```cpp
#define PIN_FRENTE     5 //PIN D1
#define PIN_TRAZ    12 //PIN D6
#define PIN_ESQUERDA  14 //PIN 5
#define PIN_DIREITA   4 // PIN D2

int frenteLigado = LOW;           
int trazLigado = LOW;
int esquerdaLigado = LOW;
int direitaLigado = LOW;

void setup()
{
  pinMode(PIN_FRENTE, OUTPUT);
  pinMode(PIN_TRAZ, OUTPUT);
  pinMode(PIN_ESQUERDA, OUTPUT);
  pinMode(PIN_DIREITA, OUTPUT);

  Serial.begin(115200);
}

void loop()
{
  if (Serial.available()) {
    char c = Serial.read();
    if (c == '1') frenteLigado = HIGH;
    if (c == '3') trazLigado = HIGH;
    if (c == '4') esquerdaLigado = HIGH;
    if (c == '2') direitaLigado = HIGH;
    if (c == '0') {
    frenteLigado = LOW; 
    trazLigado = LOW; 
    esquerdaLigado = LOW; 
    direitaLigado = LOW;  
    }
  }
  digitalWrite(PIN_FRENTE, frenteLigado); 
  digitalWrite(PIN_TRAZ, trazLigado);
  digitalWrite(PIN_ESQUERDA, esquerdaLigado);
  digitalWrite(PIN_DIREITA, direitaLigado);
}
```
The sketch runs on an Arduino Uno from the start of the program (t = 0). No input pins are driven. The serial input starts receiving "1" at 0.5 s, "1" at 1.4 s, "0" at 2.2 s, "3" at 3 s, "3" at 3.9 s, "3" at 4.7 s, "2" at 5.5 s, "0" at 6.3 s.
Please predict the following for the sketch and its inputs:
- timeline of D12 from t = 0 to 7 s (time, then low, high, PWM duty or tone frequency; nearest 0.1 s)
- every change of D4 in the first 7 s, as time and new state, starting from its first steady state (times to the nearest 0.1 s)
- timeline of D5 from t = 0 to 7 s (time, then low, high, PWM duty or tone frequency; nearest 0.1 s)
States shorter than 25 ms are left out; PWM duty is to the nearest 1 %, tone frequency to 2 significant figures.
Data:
0 s low; 3 s high; 6.3 s low
0 s low; 5.5 s high; 6.3 s low
0 s low; 0.5 s high; 2.2 s low
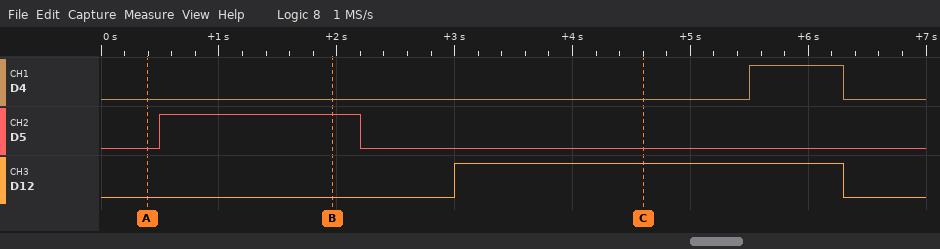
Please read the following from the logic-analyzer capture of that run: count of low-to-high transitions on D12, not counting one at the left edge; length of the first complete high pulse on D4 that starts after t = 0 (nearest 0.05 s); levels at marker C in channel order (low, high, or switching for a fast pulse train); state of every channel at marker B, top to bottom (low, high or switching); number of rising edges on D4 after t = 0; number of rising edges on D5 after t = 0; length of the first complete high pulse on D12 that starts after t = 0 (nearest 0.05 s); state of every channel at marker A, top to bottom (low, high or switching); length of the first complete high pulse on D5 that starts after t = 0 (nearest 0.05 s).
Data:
1
0.80 s
D4 low, D5 low, D12 high
D4 low, D5 high, D12 low
1
1
3.30 s
D4 low, D5 low, D12 low
1.70 s
